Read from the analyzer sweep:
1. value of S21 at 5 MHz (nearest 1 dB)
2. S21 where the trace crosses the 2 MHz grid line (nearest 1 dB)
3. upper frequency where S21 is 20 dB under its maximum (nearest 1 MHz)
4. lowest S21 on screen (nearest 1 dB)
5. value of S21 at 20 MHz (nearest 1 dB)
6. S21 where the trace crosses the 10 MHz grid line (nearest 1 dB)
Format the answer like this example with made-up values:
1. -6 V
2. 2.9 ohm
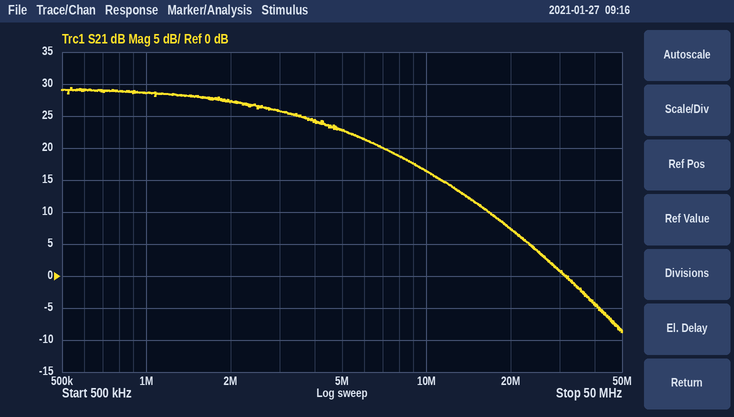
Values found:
1. 23 dB
2. 27 dB
3. 17 MHz
4. -9 dB
5. 7 dB
6. 16 dB
